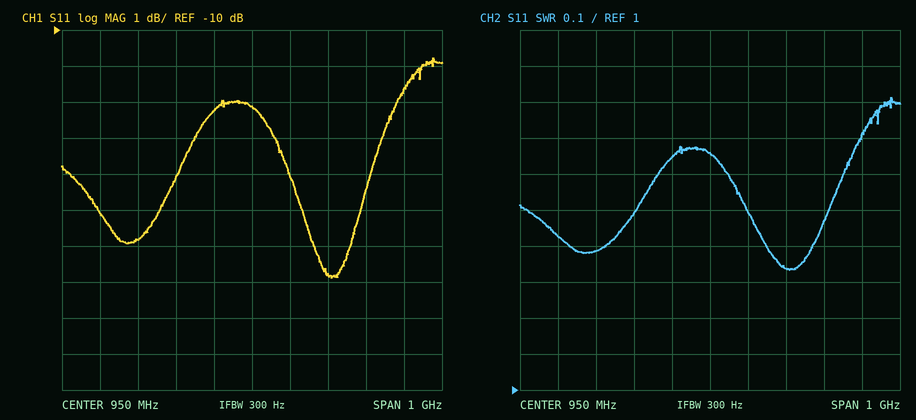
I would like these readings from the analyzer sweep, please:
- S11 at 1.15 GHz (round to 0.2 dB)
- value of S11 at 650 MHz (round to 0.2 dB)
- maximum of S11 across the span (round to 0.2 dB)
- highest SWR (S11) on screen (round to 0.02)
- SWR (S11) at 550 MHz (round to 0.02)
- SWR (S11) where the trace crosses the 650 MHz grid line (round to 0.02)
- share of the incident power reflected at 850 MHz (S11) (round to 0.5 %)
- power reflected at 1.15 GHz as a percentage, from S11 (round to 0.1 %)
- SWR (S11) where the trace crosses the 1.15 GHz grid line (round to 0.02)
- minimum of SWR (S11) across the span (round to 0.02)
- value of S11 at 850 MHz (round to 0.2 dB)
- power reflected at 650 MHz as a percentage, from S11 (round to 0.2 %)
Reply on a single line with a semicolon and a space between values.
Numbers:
-16.8 dB; -15.8 dB; -10.8 dB; 1.82; 1.42; 1.38; 6.0 %; 2.1 %; 1.34; 1.34; -12.2 dB; 2.6 %
